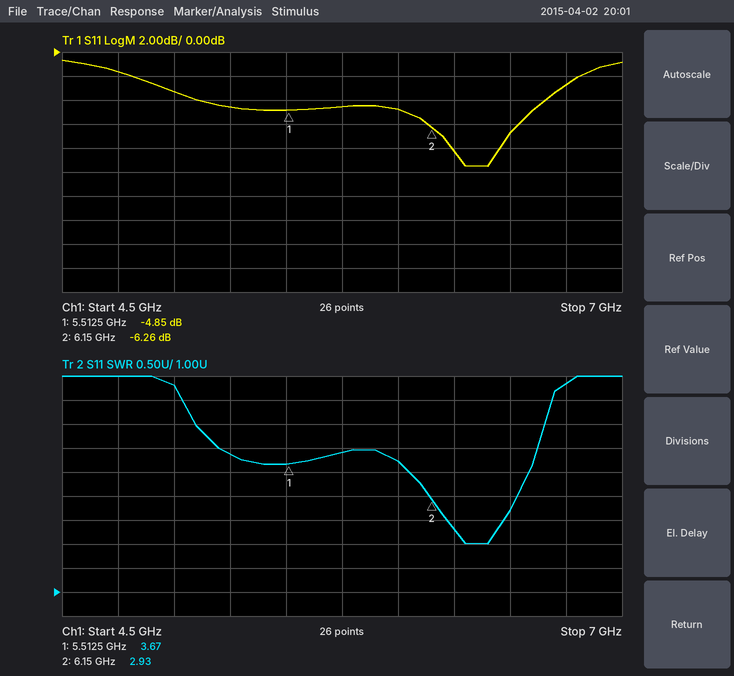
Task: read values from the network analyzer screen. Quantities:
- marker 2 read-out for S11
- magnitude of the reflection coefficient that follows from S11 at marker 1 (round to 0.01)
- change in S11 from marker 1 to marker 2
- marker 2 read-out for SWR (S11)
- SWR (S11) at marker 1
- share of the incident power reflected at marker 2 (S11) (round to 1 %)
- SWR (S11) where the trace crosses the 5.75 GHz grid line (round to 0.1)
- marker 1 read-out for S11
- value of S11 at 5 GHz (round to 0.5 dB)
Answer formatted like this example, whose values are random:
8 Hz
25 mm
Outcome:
-6.26 dB
0.57
-1.41 dB
2.93
3.67
24 %
3.9
-4.85 dB
-3.5 dB
